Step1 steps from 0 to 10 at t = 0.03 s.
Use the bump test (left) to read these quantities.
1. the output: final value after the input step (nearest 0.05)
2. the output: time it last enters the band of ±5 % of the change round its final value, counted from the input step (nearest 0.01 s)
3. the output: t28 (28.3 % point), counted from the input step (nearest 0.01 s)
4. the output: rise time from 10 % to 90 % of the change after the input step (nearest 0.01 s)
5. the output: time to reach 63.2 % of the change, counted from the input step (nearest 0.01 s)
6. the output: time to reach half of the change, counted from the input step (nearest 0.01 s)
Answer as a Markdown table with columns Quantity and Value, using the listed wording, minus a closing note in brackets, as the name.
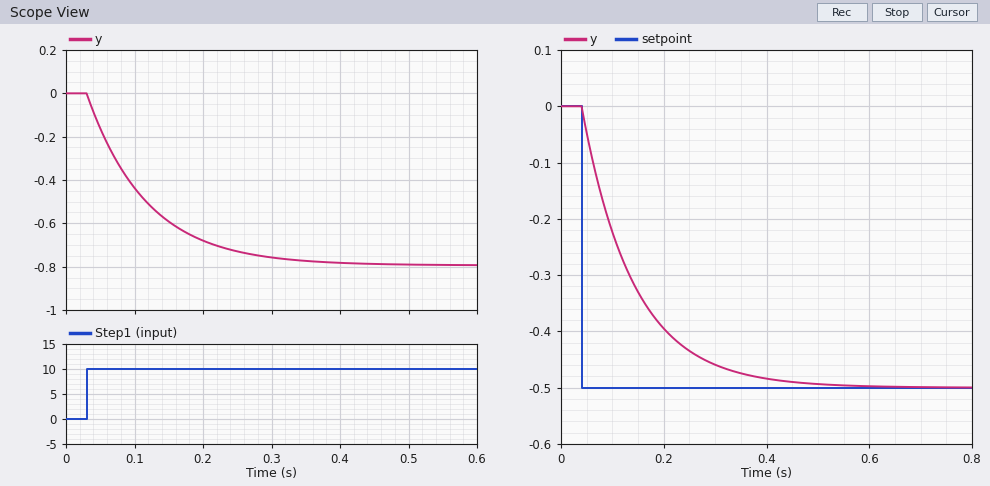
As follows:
| Quantity | Value |
|---|---|
| the output: final value after the input step | -0.80 |
| the output: time it last enters the band of ±5 % of the change round its final value, counted from the input step | 0.26 s |
| the output: t28 (28.3 % point), counted from the input step | 0.03 s |
| the output: rise time from 10 % to 90 % of the change after the input step | 0.19 s |
| the output: time to reach 63.2 % of the change, counted from the input step | 0.09 s |
| the output: time to reach half of the change, counted from the input step | 0.06 s |
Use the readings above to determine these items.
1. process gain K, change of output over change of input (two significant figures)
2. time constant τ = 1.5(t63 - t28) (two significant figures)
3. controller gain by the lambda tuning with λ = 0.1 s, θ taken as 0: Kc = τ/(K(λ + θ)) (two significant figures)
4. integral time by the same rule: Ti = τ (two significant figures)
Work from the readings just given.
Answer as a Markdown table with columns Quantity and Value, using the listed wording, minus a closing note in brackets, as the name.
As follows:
| Quantity | Value |
|---|---|
| process gain K, change of output over change of input | -0.080 |
| time constant τ = 1.5(t63 - t28) | 0.090 s |
| controller gain by the lambda tuning with λ = 0.1 s, θ taken as 0: Kc = τ/(K(λ + θ)) | -11 |
| integral time by the same rule: Ti = τ | 0.090 s |
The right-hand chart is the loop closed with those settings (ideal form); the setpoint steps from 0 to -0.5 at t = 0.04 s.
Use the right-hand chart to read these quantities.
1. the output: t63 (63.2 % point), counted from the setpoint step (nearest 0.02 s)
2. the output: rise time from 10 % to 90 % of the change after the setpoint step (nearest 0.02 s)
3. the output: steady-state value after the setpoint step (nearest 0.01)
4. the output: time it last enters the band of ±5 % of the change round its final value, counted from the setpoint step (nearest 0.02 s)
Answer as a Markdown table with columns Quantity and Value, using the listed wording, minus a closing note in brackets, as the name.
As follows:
| Quantity | Value |
|---|---|
| the output: t63 (63.2 % point), counted from the setpoint step | 0.10 s |
| the output: rise time from 10 % to 90 % of the change after the setpoint step | 0.22 s |
| the output: steady-state value after the setpoint step | -0.50 |
| the output: time it last enters the band of ±5 % of the change round its final value, counted from the setpoint step | 0.32 s |
